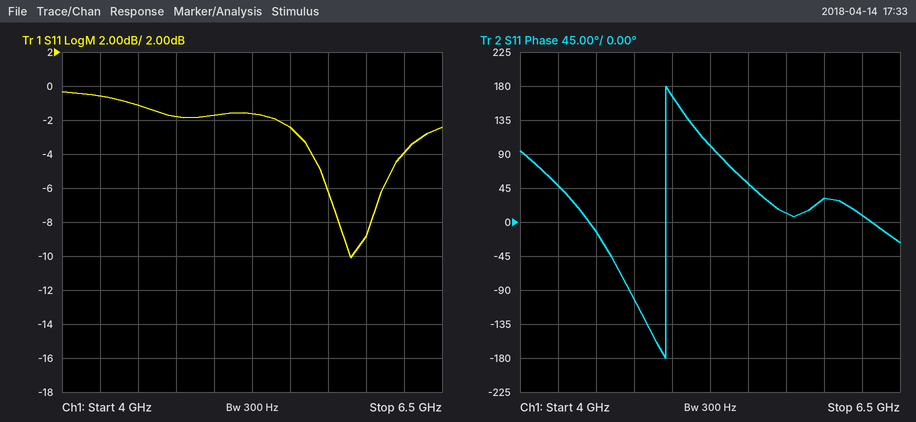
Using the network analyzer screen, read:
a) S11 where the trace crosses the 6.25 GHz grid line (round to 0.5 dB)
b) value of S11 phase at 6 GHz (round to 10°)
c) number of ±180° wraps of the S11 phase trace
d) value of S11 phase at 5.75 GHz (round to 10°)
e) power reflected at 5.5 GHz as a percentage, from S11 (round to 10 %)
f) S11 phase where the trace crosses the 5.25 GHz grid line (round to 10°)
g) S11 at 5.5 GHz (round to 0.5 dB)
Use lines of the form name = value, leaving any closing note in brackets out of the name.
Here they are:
S11 where the trace crosses the 6.25 GHz grid line = -4.0 dB
value of S11 phase at 6 GHz = 30°
number of ±180° wraps of the S11 phase trace = 1
value of S11 phase at 5.75 GHz = 10°
power reflected at 5.5 GHz as a percentage, from S11 = 60 %
S11 phase where the trace crosses the 5.25 GHz grid line = 100°
S11 at 5.5 GHz = -2.5 dB
